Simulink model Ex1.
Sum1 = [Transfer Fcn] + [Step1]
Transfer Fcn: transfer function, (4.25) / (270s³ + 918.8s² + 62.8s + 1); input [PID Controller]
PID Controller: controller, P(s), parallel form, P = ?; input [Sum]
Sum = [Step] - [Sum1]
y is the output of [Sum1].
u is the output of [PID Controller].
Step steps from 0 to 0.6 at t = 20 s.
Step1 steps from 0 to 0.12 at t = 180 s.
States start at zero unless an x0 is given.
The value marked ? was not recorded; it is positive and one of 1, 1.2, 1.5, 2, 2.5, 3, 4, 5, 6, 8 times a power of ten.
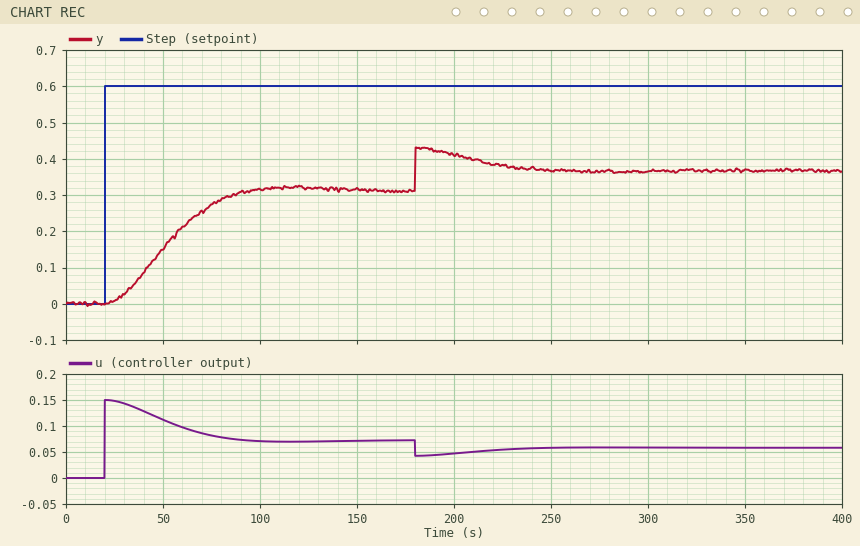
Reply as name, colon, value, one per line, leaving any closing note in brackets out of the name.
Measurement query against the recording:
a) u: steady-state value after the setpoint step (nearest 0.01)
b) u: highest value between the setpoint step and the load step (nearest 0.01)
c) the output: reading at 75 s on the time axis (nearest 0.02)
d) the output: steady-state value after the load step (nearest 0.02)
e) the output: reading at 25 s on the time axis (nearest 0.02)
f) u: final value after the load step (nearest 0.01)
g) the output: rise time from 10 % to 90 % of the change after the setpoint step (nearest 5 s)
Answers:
u: steady-state value after the setpoint step: 0.07
u: highest value between the setpoint step and the load step: 0.15
the output: reading at 75 s on the time axis: 0.28
the output: steady-state value after the load step: 0.36
the output: reading at 25 s on the time axis: 0.00
u: final value after the load step: 0.06
the output: rise time from 10 % to 90 % of the change after the setpoint step: 45 s
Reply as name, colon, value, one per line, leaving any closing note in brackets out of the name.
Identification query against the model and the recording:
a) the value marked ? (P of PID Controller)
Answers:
the value marked ?: 0.25
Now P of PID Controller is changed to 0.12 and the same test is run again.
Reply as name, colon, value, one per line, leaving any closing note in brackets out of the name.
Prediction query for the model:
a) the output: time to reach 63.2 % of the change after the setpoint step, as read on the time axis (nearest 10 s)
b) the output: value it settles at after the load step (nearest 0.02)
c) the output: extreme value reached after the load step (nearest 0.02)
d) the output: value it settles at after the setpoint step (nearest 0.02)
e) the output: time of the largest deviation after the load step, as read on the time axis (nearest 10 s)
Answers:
the output: time to reach 63.2 % of the change after the setpoint step, as read on the time axis: 70 s
the output: value it settles at after the load step: 0.28
the output: extreme value reached after the load step: 0.32
the output: value it settles at after the setpoint step: 0.20
the output: time of the largest deviation after the load step, as read on the time axis: 180 s
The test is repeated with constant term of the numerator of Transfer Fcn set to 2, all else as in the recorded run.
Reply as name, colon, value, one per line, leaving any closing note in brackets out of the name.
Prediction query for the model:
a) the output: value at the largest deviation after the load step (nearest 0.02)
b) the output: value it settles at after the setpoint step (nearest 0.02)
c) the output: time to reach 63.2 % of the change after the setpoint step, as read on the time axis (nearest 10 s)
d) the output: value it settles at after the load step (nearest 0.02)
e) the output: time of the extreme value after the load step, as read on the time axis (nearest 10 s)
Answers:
the output: value at the largest deviation after the load step: 0.32
the output: value it settles at after the setpoint step: 0.20
the output: time to reach 63.2 % of the change after the setpoint step, as read on the time axis: 70 s
the output: value it settles at after the load step: 0.28
the output: time of the extreme value after the load step, as read on the time axis: 180 s
